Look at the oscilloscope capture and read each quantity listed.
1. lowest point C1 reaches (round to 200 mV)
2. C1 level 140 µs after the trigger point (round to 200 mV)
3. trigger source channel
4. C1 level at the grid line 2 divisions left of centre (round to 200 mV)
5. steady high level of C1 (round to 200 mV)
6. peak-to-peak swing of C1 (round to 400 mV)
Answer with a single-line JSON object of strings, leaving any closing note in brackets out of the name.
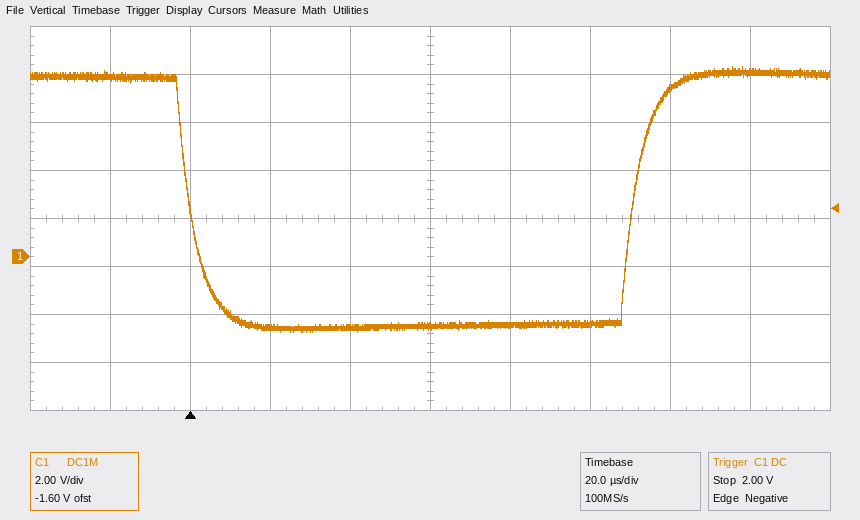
{"lowest point C1 reaches": "-3.2 V", "C1 level 140 µs after the trigger point": "7.6 V", "trigger source channel": "C1", "C1 level at the grid line 2 divisions left of centre": "-3.0 V", "steady high level of C1": "7.6 V", "peak-to-peak swing of C1": "11.2 V"}
